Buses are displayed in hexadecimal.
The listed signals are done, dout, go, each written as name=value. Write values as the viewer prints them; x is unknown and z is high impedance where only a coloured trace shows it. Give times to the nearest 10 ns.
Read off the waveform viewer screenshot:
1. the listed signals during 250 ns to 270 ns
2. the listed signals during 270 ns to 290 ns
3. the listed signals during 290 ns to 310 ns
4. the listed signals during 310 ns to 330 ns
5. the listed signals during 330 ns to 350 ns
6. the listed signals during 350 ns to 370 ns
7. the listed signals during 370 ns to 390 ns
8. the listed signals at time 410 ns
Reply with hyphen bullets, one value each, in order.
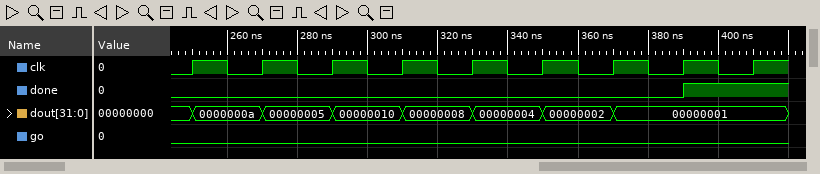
- done=0, dout=0000000a, go=0
- done=0, dout=00000005, go=0
- done=0, dout=00000010, go=0
- done=0, dout=00000008, go=0
- done=0, dout=00000004, go=0
- done=0, dout=00000002, go=0
- done=0, dout=00000001, go=0
- done=1, dout=00000001, go=0
